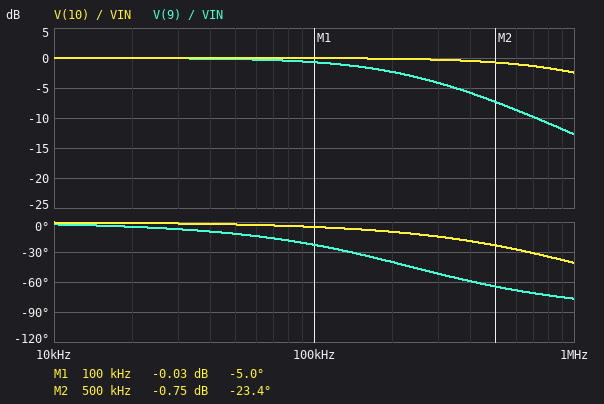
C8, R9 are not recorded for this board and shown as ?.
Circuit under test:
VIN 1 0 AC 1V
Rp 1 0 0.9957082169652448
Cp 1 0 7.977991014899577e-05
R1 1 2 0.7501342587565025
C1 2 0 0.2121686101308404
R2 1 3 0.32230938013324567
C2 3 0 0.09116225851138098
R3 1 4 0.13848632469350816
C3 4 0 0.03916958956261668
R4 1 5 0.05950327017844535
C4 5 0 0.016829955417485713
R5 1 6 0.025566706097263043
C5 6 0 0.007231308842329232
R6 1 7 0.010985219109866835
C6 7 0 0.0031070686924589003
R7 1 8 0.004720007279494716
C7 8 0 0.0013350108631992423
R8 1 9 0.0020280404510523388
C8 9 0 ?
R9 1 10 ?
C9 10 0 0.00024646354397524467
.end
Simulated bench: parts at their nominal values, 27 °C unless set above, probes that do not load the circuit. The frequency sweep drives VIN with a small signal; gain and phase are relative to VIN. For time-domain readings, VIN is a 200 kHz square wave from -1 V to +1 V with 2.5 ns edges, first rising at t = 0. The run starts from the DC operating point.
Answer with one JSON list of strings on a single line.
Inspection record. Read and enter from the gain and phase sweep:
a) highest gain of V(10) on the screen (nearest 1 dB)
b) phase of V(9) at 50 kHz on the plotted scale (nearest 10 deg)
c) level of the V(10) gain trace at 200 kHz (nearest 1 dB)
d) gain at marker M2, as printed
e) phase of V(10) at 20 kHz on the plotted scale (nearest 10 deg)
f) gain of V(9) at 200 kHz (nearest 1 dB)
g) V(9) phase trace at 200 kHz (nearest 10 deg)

["0 dB", "-10 deg", "0 dB", "-0.75 dB", "0 deg", "-2 dB", "-40 deg"]
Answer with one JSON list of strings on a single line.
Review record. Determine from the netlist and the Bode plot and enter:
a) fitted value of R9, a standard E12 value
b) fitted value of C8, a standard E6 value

["560 µΩ", "330 µF"]
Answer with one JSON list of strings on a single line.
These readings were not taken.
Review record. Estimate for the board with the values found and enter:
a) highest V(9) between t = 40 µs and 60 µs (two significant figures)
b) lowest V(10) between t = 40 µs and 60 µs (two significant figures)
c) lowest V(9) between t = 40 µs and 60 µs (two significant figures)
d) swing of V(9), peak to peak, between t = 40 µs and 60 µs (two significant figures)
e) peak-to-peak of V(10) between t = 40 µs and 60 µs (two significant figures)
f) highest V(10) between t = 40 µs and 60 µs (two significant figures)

["950 mV", "-1.0 V", "-950 mV", "1.9 V", "2.0 V", "1.0 V"]
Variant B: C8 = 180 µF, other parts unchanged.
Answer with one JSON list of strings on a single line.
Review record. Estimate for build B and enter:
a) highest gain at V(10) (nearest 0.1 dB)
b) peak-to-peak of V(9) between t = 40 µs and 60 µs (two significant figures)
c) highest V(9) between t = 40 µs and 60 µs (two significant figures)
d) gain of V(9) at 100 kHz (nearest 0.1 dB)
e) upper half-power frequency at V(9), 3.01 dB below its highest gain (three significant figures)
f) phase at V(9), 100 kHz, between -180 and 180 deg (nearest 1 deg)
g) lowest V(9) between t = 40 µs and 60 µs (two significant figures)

["0 dB", "2.0 V", "1.0 V", "-0.2 dB", "436 kHz", "-13 deg", "-1.0 V"]
